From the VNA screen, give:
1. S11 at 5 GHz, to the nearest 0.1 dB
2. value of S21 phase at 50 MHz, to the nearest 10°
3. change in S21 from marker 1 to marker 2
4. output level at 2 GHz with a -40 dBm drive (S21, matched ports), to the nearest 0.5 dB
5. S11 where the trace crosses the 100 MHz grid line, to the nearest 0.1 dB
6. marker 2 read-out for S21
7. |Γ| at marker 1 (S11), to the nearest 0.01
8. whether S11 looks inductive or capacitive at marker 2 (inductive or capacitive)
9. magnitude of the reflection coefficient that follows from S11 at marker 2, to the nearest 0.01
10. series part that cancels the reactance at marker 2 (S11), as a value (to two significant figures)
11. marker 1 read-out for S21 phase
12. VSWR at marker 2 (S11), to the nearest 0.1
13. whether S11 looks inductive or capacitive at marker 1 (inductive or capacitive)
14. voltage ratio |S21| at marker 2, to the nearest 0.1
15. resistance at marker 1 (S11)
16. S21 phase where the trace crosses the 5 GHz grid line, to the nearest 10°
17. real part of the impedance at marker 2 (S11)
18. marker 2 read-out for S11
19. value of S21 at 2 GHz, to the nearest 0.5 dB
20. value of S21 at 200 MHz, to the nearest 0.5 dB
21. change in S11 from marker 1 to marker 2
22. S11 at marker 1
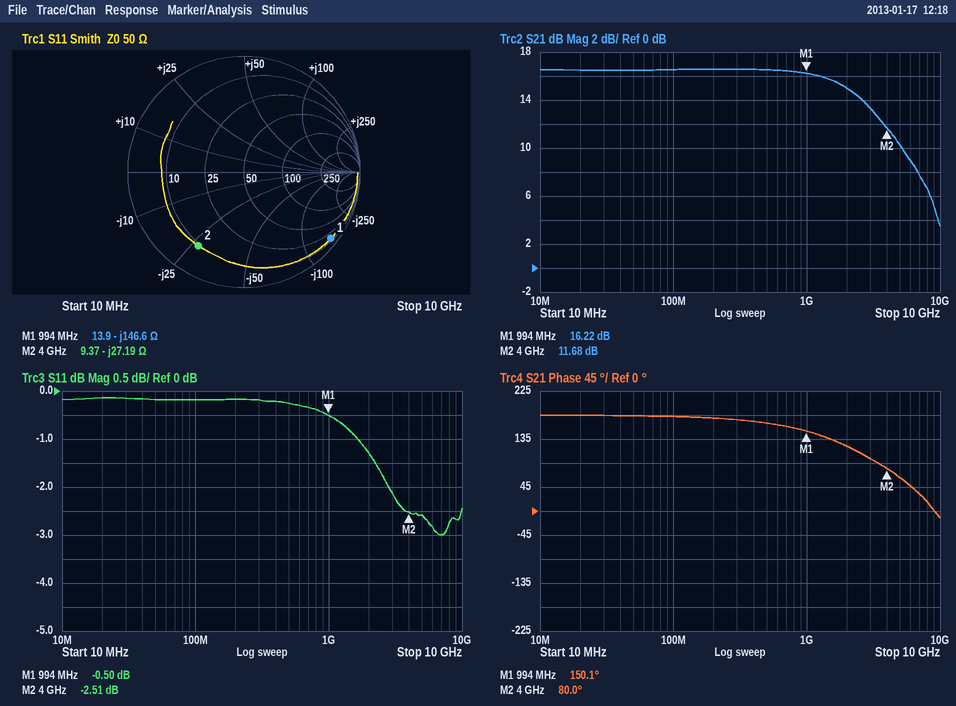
-2.6 dB
180°
-4.54 dB
-25.0 dBm
-0.2 dB
11.68 dB
0.94
capacitive
0.75
1.1 nH
150.1°
7.0
capacitive
3.8
13.9 Ω
60°
9.37 Ω
-2.51 dB
15.0 dB
16.5 dB
-2.01 dB
-0.50 dB
